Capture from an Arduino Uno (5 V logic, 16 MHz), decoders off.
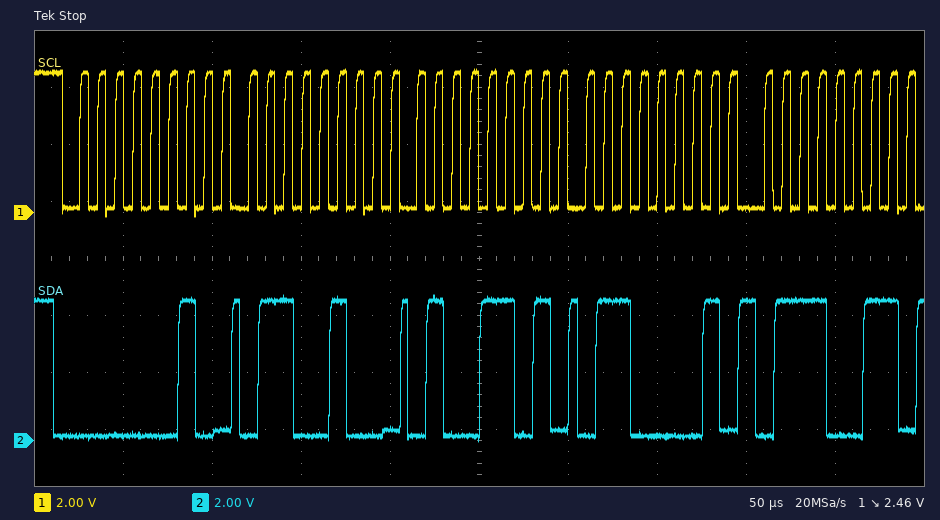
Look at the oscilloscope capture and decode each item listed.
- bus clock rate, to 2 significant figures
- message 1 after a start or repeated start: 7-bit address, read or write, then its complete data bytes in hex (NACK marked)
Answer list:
100 kHz
0x01 write: 64 4D 61 73
